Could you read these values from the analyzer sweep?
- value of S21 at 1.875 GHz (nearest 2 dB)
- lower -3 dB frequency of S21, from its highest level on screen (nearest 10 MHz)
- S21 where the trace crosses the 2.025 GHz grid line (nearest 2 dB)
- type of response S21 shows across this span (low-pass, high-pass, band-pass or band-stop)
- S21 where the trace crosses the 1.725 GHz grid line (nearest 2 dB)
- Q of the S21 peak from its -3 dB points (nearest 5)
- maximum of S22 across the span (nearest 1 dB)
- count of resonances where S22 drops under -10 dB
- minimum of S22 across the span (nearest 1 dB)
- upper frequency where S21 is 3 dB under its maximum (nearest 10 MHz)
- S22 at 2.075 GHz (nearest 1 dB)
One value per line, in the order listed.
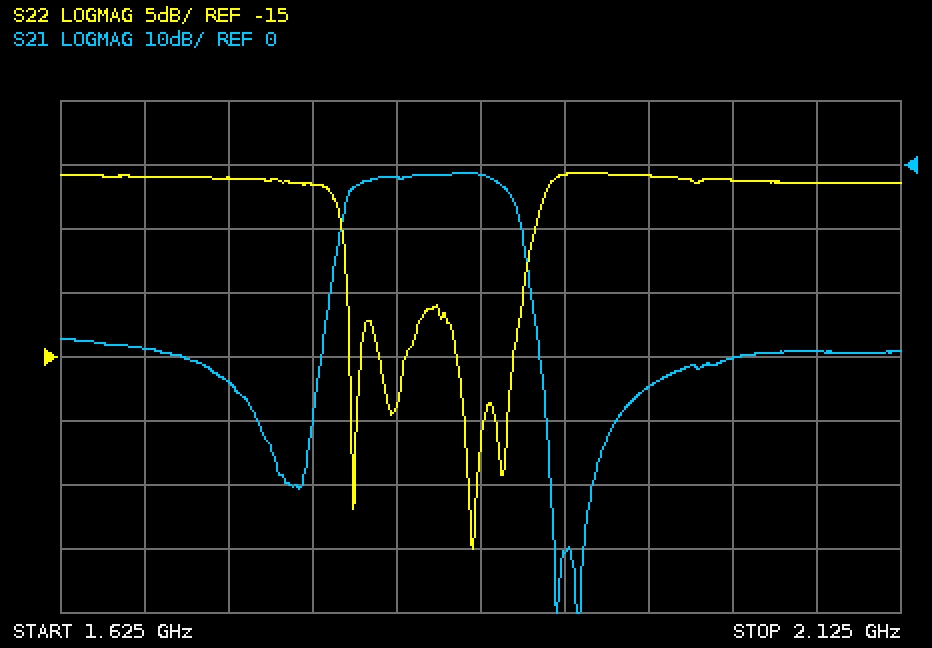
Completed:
-2 dB
1.80 GHz
-30 dB
band-pass
-34 dB
20
-1 dB
4
-30 dB
1.89 GHz
-1 dB
